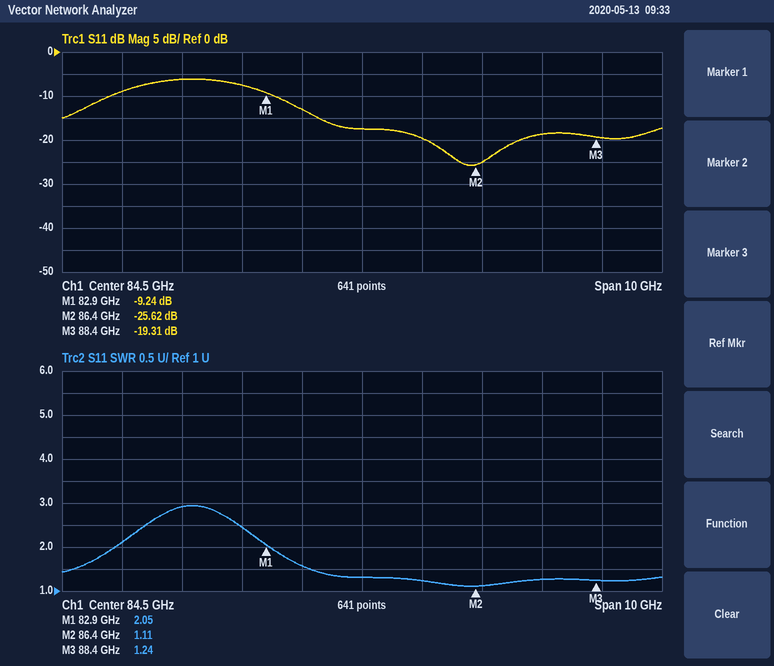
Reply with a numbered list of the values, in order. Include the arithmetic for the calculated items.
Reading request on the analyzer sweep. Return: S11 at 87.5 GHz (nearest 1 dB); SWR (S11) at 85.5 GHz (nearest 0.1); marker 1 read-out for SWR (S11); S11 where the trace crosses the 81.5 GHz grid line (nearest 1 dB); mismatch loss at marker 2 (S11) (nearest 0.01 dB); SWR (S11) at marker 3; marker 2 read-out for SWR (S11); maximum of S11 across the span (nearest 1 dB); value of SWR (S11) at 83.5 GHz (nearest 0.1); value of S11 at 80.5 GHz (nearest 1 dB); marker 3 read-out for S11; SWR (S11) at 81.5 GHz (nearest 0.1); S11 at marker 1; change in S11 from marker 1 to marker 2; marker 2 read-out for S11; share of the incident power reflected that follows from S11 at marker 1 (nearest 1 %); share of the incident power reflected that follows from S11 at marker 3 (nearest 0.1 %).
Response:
1. -19 dB
2. 1.2
3. 2.05
4. -6 dB
5. −10 log10(1 − 10^(-25.62/10)) ≈ 0.01 dB
6. 1.24
7. 1.11
8. -6 dB
9. 1.6
10. -9 dB
11. -19.31 dB
12. 2.9
13. -9.24 dB
14. -25.62 − (-9.24) = -16.38 dB
15. -25.62 dB
16. 10^(-9.24/10) ≈ 12 %
17. 10^(-19.31/10) ≈ 1.2 %
